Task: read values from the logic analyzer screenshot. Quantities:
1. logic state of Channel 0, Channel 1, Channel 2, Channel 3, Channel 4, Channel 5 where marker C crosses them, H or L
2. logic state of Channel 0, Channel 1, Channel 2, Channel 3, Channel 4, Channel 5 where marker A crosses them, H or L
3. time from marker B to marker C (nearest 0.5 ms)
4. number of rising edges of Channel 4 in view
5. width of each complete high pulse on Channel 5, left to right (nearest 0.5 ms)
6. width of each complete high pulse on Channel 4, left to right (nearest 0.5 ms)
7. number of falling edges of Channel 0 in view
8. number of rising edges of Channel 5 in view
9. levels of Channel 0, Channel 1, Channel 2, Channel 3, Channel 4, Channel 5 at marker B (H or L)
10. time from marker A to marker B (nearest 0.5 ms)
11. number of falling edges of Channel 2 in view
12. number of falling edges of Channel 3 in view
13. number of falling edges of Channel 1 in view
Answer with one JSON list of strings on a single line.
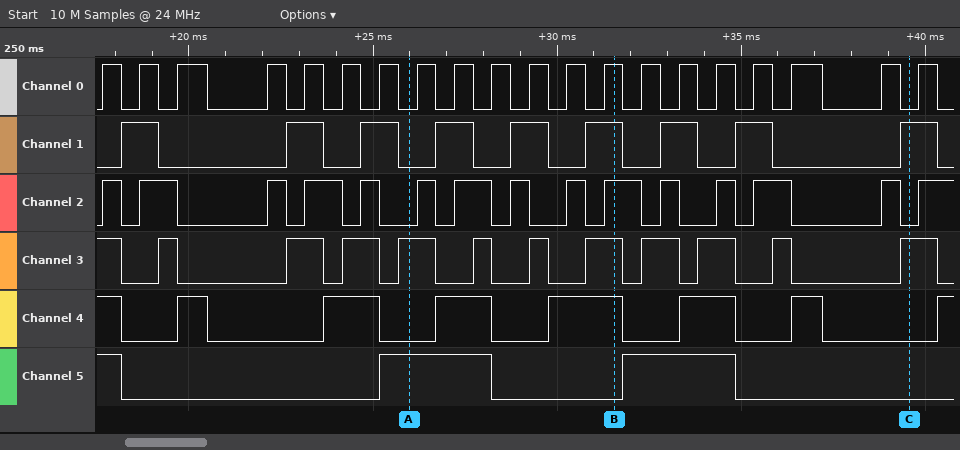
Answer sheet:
["Channel 0=L, Channel 1=H, Channel 2=L, Channel 3=H, Channel 4=L, Channel 5=L", "Channel 0=L, Channel 1=L, Channel 2=L, Channel 3=H, Channel 4=L, Channel 5=H", "8 ms", "7", "3 ms, 3 ms", "1 ms, 1.5 ms, 1.5 ms, 2 ms, 1.5 ms, 1 ms", "20", "2", "Channel 0=H, Channel 1=H, Channel 2=H, Channel 3=H, Channel 4=H, Channel 5=L", "5.5 ms", "14", "12", "9"]
